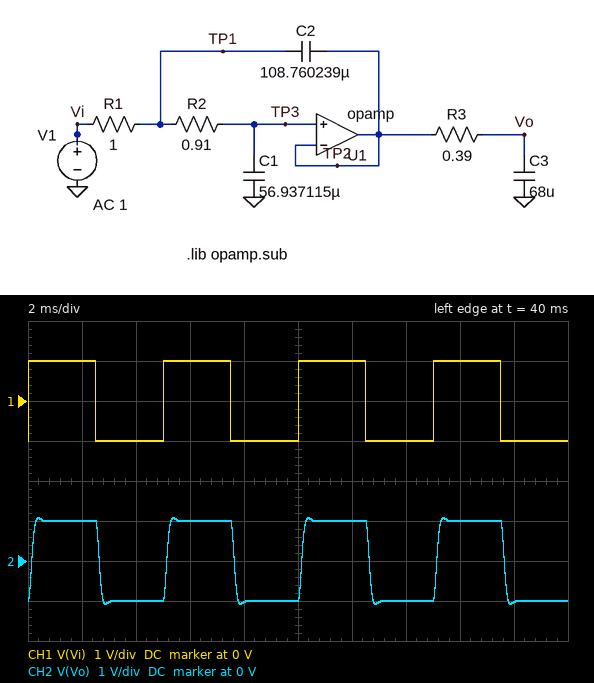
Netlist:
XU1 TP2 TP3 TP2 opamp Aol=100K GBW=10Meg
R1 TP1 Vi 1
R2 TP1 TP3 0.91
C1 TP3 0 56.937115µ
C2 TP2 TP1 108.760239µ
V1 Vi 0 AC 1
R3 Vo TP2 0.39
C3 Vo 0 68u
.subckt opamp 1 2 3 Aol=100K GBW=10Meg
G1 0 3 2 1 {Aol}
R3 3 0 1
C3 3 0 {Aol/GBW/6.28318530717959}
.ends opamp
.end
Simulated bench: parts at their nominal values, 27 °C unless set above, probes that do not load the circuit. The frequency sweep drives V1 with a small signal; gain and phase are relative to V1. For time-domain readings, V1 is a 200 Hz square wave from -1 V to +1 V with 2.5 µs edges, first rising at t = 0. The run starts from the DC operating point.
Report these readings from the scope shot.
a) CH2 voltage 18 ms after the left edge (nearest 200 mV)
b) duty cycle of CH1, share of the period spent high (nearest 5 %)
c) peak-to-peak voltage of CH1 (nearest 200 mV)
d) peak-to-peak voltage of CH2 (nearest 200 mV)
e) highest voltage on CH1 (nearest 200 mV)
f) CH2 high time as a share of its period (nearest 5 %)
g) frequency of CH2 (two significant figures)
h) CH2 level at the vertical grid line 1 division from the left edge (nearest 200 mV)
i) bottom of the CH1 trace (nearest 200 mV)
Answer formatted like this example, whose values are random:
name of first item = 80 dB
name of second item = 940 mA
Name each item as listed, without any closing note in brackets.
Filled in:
CH2 voltage 18 ms after the left edge = -1.0 V
duty cycle of CH1, share of the period spent high = 50 %
peak-to-peak voltage of CH1 = 2.0 V
peak-to-peak voltage of CH2 = 2.2 V
highest voltage on CH1 = 1.0 V
CH2 high time as a share of its period = 50 %
frequency of CH2 = 200 Hz
CH2 level at the vertical grid line 1 division from the left edge = 1.0 V
bottom of the CH1 trace = -1.0 V
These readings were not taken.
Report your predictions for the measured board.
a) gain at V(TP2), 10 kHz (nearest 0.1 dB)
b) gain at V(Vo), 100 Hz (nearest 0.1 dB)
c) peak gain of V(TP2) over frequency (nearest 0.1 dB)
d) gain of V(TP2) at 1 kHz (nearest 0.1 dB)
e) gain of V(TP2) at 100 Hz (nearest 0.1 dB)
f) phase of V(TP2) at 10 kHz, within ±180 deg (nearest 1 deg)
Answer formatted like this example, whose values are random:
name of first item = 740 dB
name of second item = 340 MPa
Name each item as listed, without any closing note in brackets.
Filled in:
gain at V(TP2), 10 kHz = -27.0 dB
gain at V(Vo), 100 Hz = 0 dB
peak gain of V(TP2) over frequency = 0 dB
gain of V(TP2) at 1 kHz = -0.3 dB
gain of V(TP2) at 100 Hz = 0 dB
phase of V(TP2) at 10 kHz, within ±180 deg = -162 deg
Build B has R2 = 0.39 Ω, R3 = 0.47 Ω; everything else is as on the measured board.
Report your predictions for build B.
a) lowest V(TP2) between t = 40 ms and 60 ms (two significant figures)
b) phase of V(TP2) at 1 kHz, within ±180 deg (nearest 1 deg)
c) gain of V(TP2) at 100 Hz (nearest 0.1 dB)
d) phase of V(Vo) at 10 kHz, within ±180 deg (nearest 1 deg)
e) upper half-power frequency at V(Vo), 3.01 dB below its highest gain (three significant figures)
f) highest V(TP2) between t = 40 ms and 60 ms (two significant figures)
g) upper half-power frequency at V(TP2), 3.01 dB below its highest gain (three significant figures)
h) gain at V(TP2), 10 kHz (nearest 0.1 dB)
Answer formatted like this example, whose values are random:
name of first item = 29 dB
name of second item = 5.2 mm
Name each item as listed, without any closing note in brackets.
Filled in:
lowest V(TP2) between t = 40 ms and 60 ms = -1.0 V
phase of V(TP2) at 1 kHz, within ±180 deg = -29 deg
gain of V(TP2) at 100 Hz = 0 dB
phase of V(Vo) at 10 kHz, within ±180 deg = 147 deg
upper half-power frequency at V(Vo), 3.01 dB below its highest gain = 2.40 kHz
highest V(TP2) between t = 40 ms and 60 ms = 1.0 V
upper half-power frequency at V(TP2), 3.01 dB below its highest gain = 2.80 kHz
gain at V(TP2), 10 kHz = -19.9 dB
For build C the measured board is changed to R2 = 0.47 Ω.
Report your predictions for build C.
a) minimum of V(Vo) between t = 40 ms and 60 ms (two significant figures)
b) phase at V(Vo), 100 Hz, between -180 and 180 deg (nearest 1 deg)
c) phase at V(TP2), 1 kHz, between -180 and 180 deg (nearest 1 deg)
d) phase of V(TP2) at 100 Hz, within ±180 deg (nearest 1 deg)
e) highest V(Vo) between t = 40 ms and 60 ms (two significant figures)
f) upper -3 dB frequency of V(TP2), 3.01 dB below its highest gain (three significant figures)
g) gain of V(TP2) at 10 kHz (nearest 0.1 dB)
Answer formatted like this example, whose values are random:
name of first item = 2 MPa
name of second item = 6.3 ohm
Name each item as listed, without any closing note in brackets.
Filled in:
minimum of V(Vo) between t = 40 ms and 60 ms = -1.0 V
phase at V(Vo), 100 Hz, between -180 and 180 deg = -4 deg
phase at V(TP2), 1 kHz, between -180 and 180 deg = -31 deg
phase of V(TP2) at 100 Hz, within ±180 deg = -3 deg
highest V(Vo) between t = 40 ms and 60 ms = 1.0 V
upper -3 dB frequency of V(TP2), 3.01 dB below its highest gain = 2.67 kHz
gain of V(TP2) at 10 kHz = -21.4 dB
